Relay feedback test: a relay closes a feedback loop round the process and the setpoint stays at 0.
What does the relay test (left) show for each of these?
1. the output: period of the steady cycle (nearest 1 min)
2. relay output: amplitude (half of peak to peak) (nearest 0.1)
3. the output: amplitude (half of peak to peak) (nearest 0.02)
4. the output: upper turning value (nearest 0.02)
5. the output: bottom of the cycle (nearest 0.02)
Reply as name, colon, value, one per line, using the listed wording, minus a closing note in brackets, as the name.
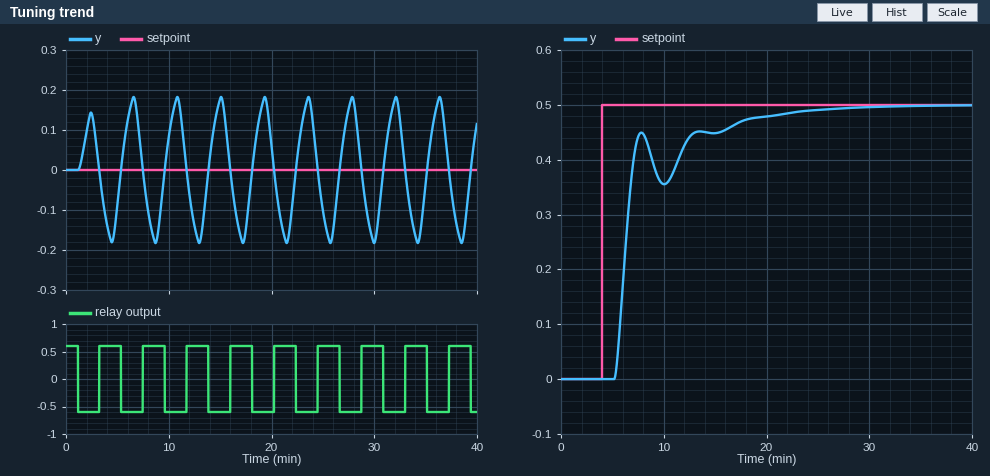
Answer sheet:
the output: period of the steady cycle: 4 min
relay output: amplitude (half of peak to peak): 0.6
the output: amplitude (half of peak to peak): 0.18
the output: upper turning value: 0.18
the output: bottom of the cycle: -0.18
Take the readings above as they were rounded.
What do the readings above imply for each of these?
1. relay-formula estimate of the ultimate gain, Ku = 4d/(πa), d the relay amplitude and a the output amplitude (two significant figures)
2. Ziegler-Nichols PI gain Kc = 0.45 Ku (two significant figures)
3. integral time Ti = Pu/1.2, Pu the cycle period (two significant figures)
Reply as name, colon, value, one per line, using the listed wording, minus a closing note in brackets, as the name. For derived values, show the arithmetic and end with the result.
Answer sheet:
relay-formula estimate of the ultimate gain, Ku = 4d/(πa), d the relay amplitude and a the output amplitude: 4 × 0.6 / (π × 0.18) = 4.2
Ziegler-Nichols PI gain Kc = 0.45 Ku: 0.45 × 4.2 = 1.9
integral time Ti = Pu/1.2, Pu the cycle period: 4 / 1.2 = 3.3 min
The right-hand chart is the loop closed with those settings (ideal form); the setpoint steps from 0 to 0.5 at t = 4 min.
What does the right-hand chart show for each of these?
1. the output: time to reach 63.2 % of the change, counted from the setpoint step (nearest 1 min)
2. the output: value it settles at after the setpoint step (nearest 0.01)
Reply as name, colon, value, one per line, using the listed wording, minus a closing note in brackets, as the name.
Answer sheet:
the output: time to reach 63.2 % of the change, counted from the setpoint step: 3 min
the output: value it settles at after the setpoint step: 0.50
